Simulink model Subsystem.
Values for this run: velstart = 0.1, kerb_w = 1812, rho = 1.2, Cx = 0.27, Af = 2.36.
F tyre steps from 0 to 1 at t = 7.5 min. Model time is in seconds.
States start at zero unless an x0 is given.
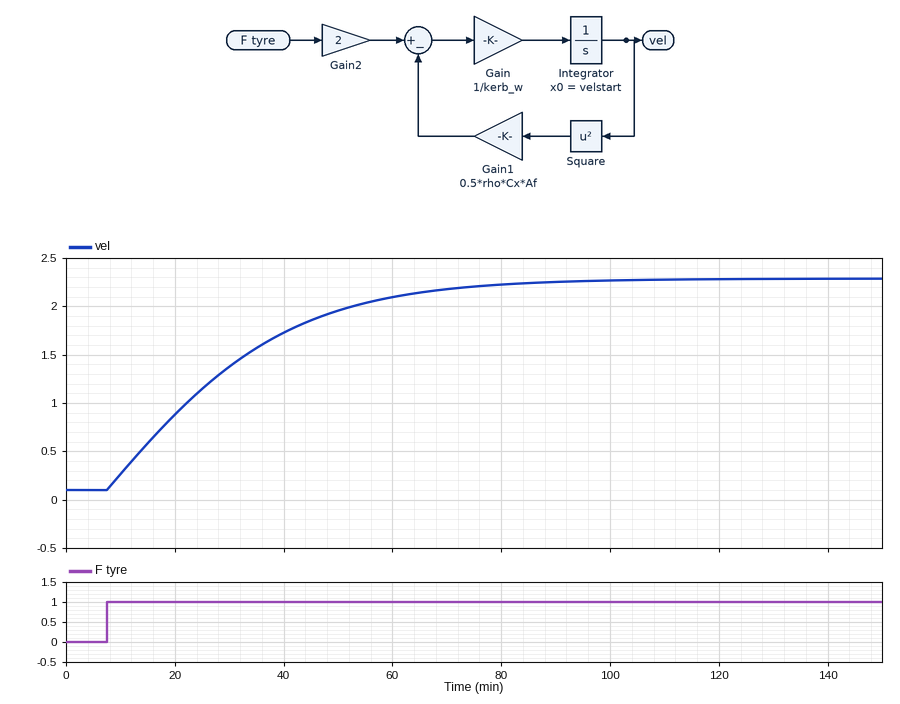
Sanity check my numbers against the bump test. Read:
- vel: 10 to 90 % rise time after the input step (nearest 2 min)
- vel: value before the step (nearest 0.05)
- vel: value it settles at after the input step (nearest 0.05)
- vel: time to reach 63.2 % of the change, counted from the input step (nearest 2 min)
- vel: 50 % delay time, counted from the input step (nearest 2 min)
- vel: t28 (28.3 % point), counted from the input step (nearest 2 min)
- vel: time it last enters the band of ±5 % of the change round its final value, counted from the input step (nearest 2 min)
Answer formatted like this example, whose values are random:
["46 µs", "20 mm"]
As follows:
["46 min", "0.10", "2.30", "26 min", "18 min", "10 min", "62 min"]
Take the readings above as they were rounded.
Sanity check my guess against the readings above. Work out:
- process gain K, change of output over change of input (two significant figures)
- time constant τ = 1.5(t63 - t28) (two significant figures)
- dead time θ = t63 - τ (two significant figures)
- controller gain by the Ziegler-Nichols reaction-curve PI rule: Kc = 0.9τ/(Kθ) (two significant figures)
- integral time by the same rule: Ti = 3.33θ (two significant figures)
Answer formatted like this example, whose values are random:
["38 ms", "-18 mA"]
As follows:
["2.2", "24 min", "2.0 min", "4.9", "6.7 min"]
